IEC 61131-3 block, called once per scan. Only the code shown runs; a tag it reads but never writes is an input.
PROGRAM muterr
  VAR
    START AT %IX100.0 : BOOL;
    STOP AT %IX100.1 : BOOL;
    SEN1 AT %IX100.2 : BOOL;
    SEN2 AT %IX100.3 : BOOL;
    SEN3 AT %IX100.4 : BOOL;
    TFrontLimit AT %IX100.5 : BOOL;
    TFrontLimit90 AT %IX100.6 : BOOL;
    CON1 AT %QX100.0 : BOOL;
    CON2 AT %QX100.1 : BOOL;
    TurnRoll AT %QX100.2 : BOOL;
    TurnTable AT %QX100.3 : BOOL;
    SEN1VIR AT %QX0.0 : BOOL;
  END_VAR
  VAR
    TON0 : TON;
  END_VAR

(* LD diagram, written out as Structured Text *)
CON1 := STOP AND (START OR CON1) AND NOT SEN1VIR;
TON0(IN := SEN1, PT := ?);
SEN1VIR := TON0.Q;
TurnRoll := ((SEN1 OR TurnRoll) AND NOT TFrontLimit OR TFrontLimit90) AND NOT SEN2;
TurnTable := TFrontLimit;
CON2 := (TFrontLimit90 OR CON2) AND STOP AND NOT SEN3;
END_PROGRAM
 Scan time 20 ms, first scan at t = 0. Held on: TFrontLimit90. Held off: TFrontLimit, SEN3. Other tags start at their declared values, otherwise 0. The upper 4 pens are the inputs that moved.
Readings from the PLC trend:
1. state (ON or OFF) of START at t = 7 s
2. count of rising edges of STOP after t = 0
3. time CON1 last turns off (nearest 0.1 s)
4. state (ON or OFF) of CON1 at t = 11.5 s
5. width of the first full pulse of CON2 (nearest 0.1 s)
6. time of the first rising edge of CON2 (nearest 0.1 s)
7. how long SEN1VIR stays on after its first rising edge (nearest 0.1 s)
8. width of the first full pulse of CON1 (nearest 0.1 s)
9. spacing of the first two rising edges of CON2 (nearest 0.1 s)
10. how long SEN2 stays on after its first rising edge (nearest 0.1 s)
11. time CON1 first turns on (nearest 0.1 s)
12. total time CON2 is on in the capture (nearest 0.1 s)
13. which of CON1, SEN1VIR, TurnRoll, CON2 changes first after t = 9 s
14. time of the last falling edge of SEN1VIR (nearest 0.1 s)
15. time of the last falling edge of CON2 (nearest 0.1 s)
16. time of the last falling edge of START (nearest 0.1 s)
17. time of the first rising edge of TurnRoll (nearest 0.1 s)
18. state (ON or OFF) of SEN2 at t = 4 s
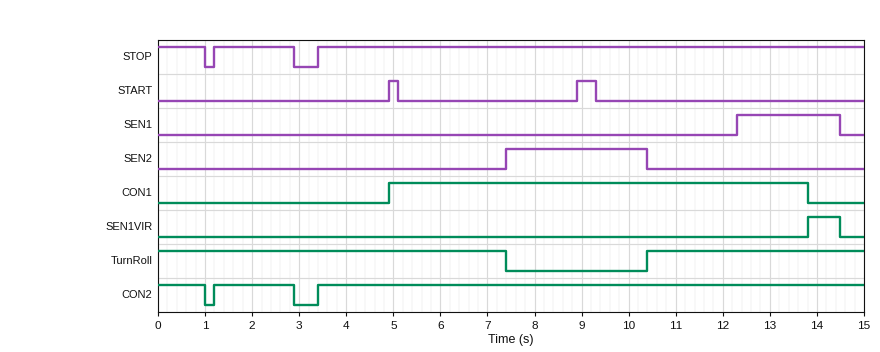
OFF
2
13.8 s
ON
1.7 s
1.2 s
0.7 s
8.9 s
2.2 s
3.0 s
4.9 s
14.3 s
TurnRoll
14.5 s
2.9 s
9.3 s
10.4 s
OFF
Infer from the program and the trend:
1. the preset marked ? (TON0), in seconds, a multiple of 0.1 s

1.5 s
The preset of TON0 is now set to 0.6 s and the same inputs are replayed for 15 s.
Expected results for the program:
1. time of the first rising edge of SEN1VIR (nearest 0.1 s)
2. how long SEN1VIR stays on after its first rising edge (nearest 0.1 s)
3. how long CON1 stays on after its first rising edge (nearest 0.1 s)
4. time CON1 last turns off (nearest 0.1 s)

12.9 s
1.6 s
8.0 s
12.9 s
